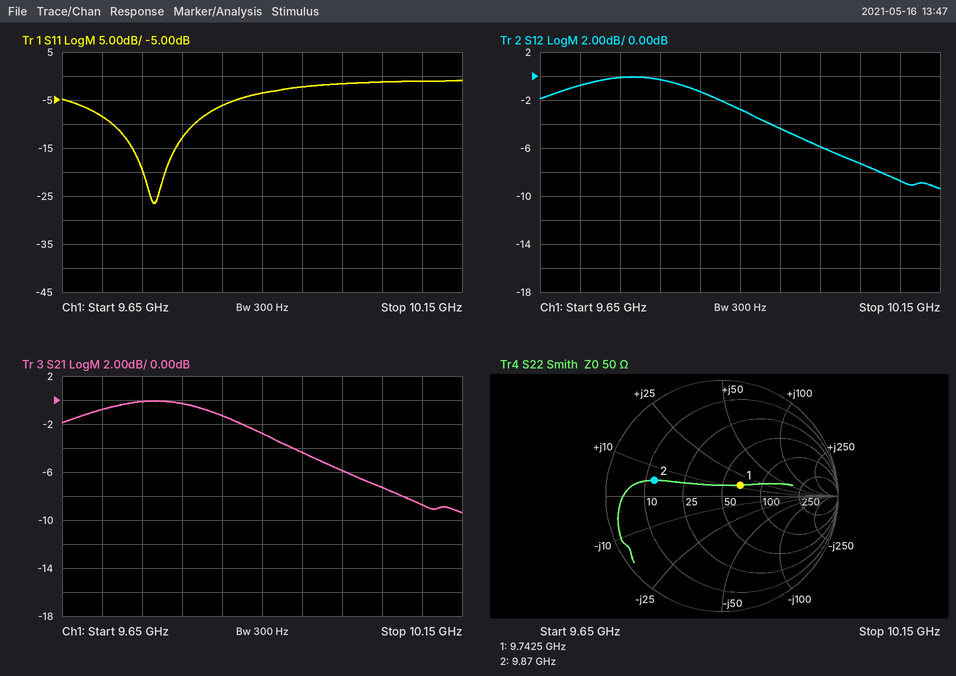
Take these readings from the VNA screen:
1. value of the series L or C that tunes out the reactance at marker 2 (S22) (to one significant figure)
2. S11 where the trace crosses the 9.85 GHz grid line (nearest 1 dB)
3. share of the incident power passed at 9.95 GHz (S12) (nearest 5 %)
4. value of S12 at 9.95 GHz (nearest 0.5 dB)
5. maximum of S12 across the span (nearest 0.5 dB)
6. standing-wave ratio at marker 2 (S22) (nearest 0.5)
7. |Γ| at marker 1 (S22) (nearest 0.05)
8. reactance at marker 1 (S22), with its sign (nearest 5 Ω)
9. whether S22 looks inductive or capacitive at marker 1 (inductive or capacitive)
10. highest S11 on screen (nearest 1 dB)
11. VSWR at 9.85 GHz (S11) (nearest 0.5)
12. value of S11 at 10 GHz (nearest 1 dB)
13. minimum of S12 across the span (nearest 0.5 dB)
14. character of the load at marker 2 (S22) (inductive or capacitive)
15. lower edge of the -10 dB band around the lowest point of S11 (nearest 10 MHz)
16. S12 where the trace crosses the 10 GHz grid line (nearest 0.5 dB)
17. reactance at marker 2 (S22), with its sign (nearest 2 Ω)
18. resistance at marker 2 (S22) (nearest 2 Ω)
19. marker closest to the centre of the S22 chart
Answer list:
3 pF
-6 dB
35 %
-4.5 dB
0.0 dB
4.0
0.20
+15 Ω
inductive
-1 dB
3.0
-2 dB
-9.5 dB
inductive
9.71 GHz
-6.0 dB
+6 Ω
12 Ω
marker 1
